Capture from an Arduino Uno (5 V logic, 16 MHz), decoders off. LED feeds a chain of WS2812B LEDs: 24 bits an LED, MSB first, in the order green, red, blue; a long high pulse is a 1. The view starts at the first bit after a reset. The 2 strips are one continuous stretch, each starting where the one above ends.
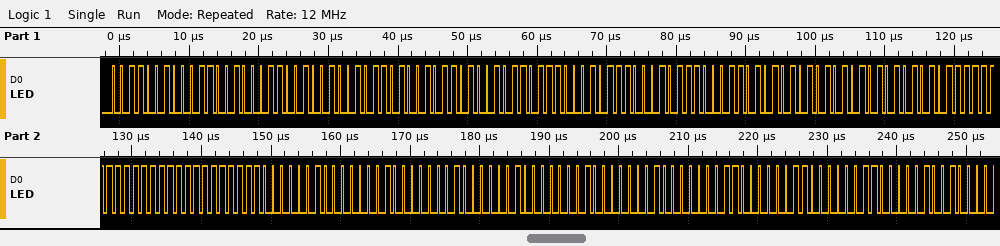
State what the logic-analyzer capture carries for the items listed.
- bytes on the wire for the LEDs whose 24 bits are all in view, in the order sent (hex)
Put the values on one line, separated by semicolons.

32 32 32 4B 4B 4B 71 71 71 AA AA AA FF FF FF 02 02 02 04 04 04 06 06 06
